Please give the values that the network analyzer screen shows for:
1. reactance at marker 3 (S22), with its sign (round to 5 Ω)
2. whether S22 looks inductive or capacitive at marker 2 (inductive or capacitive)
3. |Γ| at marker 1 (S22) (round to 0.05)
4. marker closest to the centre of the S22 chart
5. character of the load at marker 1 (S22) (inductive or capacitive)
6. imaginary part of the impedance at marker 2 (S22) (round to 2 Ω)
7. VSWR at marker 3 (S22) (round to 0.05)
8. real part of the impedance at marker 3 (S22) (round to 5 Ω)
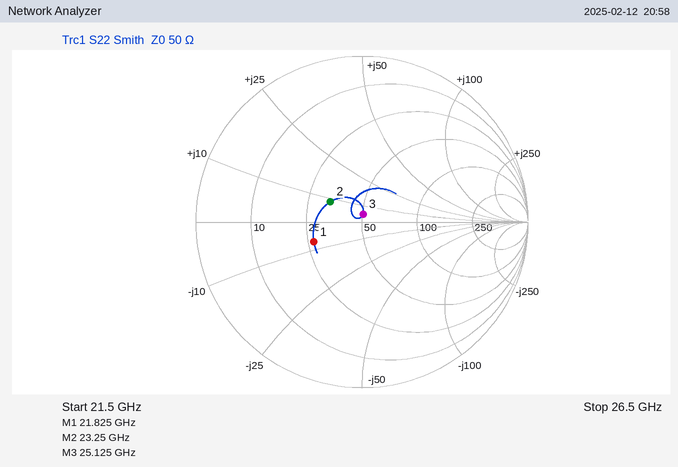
+5 Ω
inductive
0.30
marker 3
capacitive
+8 Ω
1.10
50 Ω
